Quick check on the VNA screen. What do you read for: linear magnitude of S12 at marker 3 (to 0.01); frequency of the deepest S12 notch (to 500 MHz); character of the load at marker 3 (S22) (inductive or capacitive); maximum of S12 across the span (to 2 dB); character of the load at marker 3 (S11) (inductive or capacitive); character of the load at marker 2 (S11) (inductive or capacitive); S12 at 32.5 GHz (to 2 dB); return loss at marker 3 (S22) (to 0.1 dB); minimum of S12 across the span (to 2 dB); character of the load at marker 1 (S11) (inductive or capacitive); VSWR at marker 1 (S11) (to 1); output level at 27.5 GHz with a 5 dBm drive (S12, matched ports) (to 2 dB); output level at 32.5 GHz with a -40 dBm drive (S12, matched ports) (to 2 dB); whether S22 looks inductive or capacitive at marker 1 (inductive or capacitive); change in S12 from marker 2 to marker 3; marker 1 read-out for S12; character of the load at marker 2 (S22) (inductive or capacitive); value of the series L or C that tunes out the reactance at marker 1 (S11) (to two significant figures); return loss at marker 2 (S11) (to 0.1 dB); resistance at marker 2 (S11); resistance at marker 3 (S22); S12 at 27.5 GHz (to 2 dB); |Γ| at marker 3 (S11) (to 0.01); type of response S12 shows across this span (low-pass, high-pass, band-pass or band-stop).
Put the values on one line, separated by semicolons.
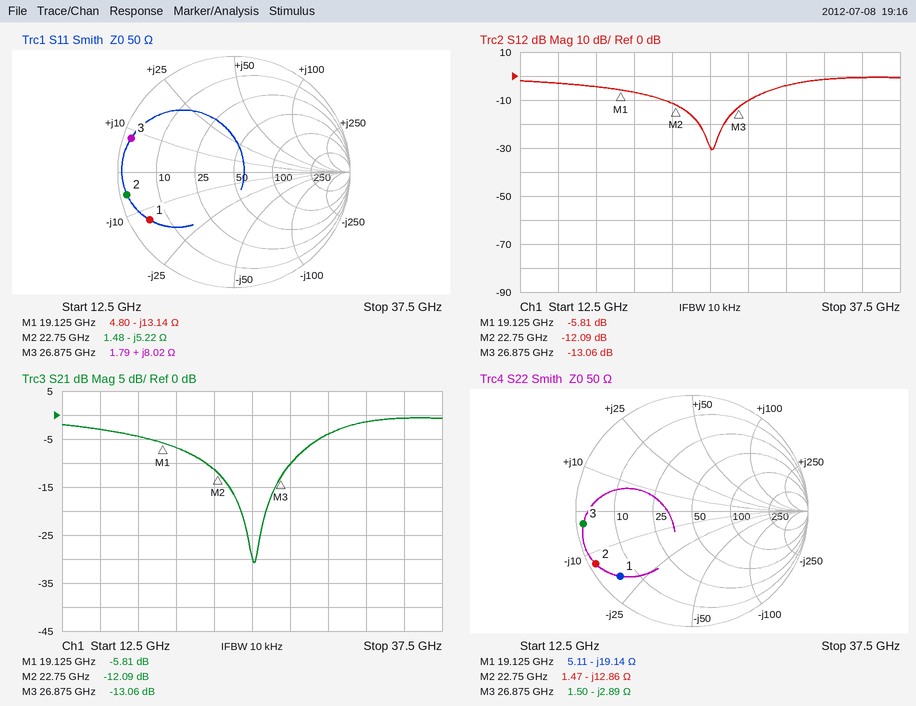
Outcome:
0.22; 25.0 GHz; capacitive; 0 dB; inductive; capacitive; -2 dB; 0.5 dB; -30 dB; capacitive; 11; -6 dBm; -42 dBm; capacitive; -0.97 dB; -5.81 dB; capacitive; 110 pH; 0.5 dB; 1.48 Ω; 1.50 Ω; -10 dB; 0.93; band-stop
